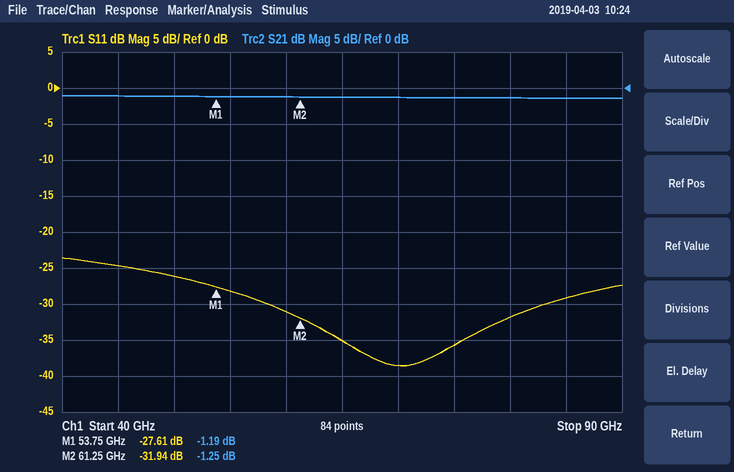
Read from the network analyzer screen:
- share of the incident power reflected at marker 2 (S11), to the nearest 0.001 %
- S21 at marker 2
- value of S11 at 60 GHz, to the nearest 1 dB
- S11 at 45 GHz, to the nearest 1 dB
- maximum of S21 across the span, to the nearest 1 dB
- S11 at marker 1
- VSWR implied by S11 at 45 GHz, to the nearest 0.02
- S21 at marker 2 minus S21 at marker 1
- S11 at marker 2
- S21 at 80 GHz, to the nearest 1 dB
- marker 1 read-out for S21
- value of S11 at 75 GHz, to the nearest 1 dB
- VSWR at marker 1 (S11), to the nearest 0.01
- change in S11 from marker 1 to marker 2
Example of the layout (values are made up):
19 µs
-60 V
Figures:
0.064 %
-1.25 dB
-31 dB
-25 dB
-1 dB
-27.61 dB
1.12
-0.06 dB
-31.94 dB
-1 dB
-1.19 dB
-36 dB
1.09
-4.33 dB
